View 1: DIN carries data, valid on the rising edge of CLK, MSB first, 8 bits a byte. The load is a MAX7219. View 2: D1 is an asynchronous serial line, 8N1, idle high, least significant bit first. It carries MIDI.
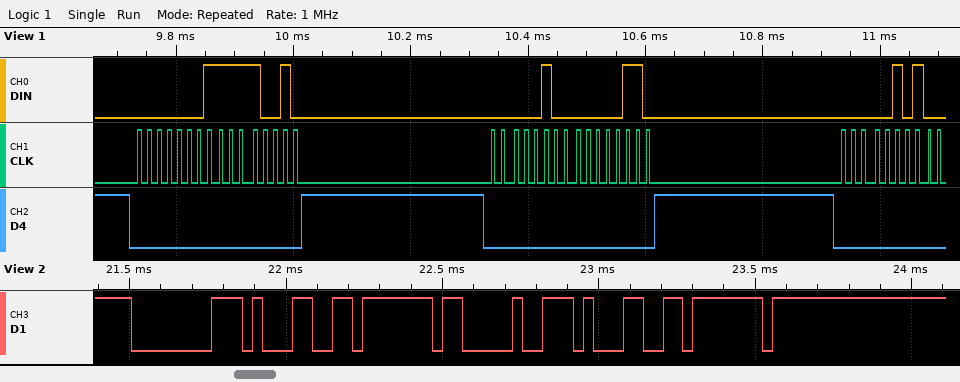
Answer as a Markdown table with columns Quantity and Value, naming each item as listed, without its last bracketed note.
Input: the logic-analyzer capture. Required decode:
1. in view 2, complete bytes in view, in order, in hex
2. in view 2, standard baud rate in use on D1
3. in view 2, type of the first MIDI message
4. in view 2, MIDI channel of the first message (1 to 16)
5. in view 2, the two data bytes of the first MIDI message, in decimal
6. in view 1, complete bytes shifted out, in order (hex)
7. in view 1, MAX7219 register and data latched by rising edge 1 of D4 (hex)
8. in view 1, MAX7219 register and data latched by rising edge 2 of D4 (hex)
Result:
| Quantity | Value |
|---|---|
| in view 2, complete bytes in view, in order, in hex | 80 31 7F 90 31 7F |
| in view 2, standard baud rate in use on D1 | 31250 baud |
| in view 2, type of the first MIDI message | Note Off |
| in view 2, MIDI channel of the first message | 1 |
| in view 2, the two data bytes of the first MIDI message, in decimal | 49, 127 |
| in view 1, complete bytes shifted out, in order | 0x01 0xF2 0x04 0x06 0x05 |
| in view 1, MAX7219 register and data latched by rising edge 1 of D4 | register 0x1, data 0xF2 |
| in view 1, MAX7219 register and data latched by rising edge 2 of D4 | register 0x4, data 0x06 |
